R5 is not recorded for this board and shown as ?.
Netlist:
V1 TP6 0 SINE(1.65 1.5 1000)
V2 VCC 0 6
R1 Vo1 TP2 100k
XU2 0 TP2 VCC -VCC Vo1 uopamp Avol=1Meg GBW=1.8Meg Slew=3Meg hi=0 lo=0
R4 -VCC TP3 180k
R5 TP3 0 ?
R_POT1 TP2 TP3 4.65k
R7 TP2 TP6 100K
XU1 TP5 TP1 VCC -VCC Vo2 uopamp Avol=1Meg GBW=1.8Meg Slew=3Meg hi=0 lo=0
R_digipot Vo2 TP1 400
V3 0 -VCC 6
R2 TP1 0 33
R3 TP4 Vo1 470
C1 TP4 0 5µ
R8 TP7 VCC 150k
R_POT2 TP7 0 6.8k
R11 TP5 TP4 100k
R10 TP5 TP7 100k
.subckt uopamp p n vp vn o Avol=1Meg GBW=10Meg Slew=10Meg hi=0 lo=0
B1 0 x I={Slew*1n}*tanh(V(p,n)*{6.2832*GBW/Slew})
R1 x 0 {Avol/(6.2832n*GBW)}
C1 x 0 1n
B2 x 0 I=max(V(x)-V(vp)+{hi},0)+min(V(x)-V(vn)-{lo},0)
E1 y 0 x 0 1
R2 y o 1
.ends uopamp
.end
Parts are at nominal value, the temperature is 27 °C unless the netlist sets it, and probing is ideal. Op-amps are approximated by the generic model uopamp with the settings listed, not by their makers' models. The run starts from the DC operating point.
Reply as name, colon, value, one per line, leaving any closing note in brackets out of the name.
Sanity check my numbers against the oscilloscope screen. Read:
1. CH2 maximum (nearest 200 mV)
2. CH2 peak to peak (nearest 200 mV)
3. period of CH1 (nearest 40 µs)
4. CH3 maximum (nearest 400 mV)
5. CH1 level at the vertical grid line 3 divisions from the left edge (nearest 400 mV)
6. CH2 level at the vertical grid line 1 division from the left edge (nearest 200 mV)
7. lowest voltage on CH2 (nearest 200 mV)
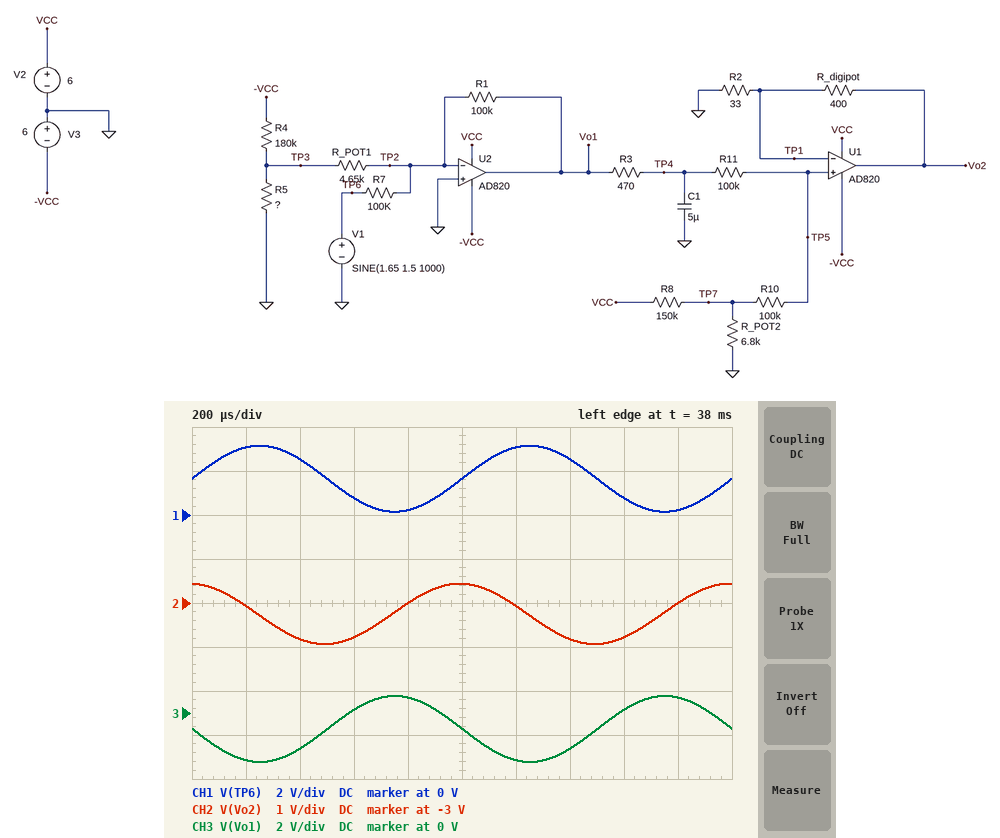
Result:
CH2 maximum: -2.6 V
CH2 peak to peak: 1.4 V
period of CH1: 1.00 ms
CH3 maximum: 800 mV
CH1 level at the vertical grid line 3 divisions from the left edge: 800 mV
CH2 level at the vertical grid line 1 division from the left edge: -3.0 V
lowest voltage on CH2: -4.0 V
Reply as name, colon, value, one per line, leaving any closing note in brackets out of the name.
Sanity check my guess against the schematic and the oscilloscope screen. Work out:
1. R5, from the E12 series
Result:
R5, from the E12 series: 1.8 kΩ
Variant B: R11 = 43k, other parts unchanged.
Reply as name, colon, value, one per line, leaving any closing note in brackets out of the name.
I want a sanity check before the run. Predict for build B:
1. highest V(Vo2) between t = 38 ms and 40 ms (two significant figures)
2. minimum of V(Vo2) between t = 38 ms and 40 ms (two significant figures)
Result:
highest V(Vo2) between t = 38 ms and 40 ms: -4.8 V
minimum of V(Vo2) between t = 38 ms and 40 ms: -6.0 V
